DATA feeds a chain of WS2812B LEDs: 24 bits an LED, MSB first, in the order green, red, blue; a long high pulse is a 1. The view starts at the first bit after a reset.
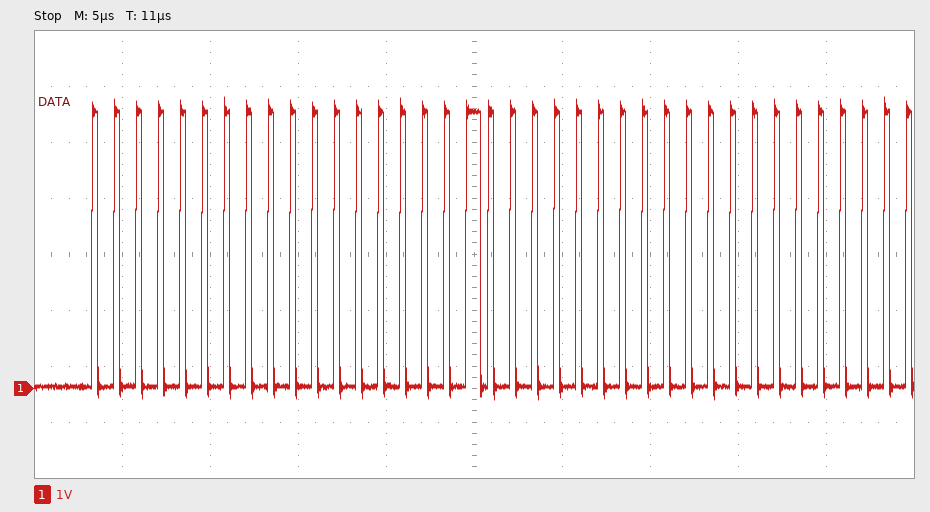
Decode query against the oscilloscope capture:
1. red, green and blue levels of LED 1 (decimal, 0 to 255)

0, 0, 64
